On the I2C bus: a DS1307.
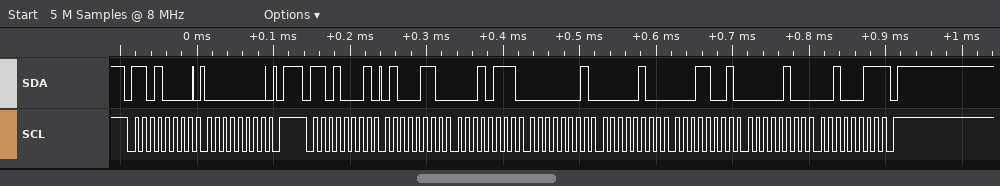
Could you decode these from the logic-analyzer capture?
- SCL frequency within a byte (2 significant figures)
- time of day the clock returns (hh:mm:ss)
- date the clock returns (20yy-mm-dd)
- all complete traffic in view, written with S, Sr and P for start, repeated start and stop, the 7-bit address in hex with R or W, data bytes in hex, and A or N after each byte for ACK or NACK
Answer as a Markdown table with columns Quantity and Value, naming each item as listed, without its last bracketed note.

| Quantity | Value |
|---|---|
| SCL frequency within a byte | 100 kHz |
| time of day the clock returns | 01:17:46 |
| date the clock returns | 2023-04-19 |
| all complete traffic in view, written with S, Sr and P for start, repeated start and stop, the 7-bit address in hex with R or W, data bytes in hex, and A or N after each byte for ACK or NACK | S 68W A 00 A P S 68R A 46 A 17 A 01 A 04 A 19 A 04 A 23 N P |
